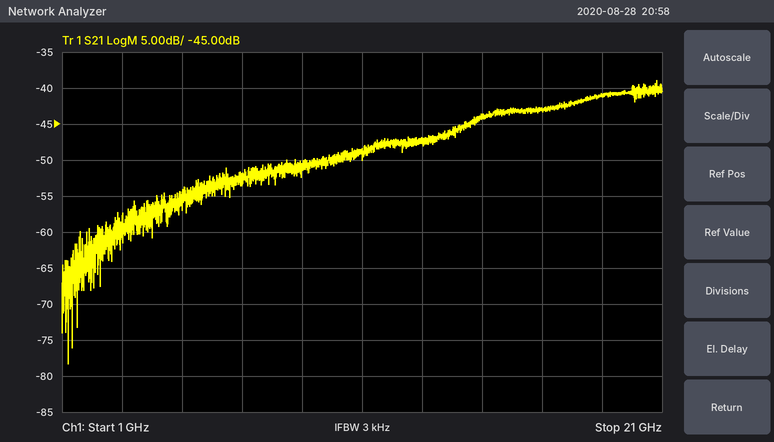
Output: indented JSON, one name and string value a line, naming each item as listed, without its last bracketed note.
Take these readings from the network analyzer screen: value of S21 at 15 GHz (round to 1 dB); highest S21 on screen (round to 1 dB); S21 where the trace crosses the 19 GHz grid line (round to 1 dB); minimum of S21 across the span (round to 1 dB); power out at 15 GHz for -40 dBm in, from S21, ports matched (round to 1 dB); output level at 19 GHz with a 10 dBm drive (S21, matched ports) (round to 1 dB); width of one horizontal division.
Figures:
{
  "value of S21 at 15 GHz": "-44 dB",
  "highest S21 on screen": "-39 dB",
  "S21 where the trace crosses the 19 GHz grid line": "-41 dB",
  "minimum of S21 across the span": "-78 dB",
  "power out at 15 GHz for -40 dBm in, from S21, ports matched": "-84 dBm",
  "output level at 19 GHz with a 10 dBm drive (S21, matched ports)": "-31 dBm",
  "width of one horizontal division": "2 GHz"
}
